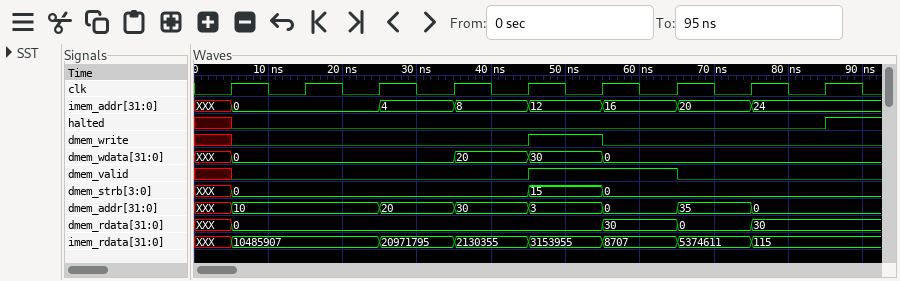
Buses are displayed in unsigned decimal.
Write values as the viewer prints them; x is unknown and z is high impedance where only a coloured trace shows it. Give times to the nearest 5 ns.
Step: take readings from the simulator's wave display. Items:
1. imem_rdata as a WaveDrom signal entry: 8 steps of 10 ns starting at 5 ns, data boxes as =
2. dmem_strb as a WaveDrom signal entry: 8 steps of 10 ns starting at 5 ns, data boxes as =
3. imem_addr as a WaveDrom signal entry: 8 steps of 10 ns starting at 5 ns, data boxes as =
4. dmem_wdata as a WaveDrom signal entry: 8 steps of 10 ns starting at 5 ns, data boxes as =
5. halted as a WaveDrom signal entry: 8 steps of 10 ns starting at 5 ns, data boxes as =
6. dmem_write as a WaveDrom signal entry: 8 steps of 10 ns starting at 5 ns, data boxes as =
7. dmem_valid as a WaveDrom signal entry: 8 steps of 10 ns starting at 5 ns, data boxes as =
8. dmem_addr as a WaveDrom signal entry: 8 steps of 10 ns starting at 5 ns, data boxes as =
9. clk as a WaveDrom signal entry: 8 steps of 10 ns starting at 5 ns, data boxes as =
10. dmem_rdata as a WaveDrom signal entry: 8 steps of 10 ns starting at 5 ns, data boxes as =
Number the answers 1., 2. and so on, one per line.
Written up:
1. {name: 'imem_rdata', wave: '=.======', data: '10485907 20971795 2130355 3153955 8707 5374611 115'}
2. {name: 'dmem_strb', wave: '=...==..', data: '0 15 0'}
3. {name: 'imem_addr', wave: '=.======', data: '0 4 8 12 16 20 24'}
4. {name: 'dmem_wdata', wave: '=..===..', data: '0 20 30 0'}
5. {name: 'halted', wave: '0.......'}
6. {name: 'dmem_write', wave: '0...10..'}
7. {name: 'dmem_valid', wave: '0...1.0.'}
8. {name: 'dmem_addr', wave: '=.======', data: '10 20 30 3 0 35 0'}
9. {name: 'clk', wave: 'p.......'}
10. {name: 'dmem_rdata', wave: '=....===', data: '0 30 0 30'}
